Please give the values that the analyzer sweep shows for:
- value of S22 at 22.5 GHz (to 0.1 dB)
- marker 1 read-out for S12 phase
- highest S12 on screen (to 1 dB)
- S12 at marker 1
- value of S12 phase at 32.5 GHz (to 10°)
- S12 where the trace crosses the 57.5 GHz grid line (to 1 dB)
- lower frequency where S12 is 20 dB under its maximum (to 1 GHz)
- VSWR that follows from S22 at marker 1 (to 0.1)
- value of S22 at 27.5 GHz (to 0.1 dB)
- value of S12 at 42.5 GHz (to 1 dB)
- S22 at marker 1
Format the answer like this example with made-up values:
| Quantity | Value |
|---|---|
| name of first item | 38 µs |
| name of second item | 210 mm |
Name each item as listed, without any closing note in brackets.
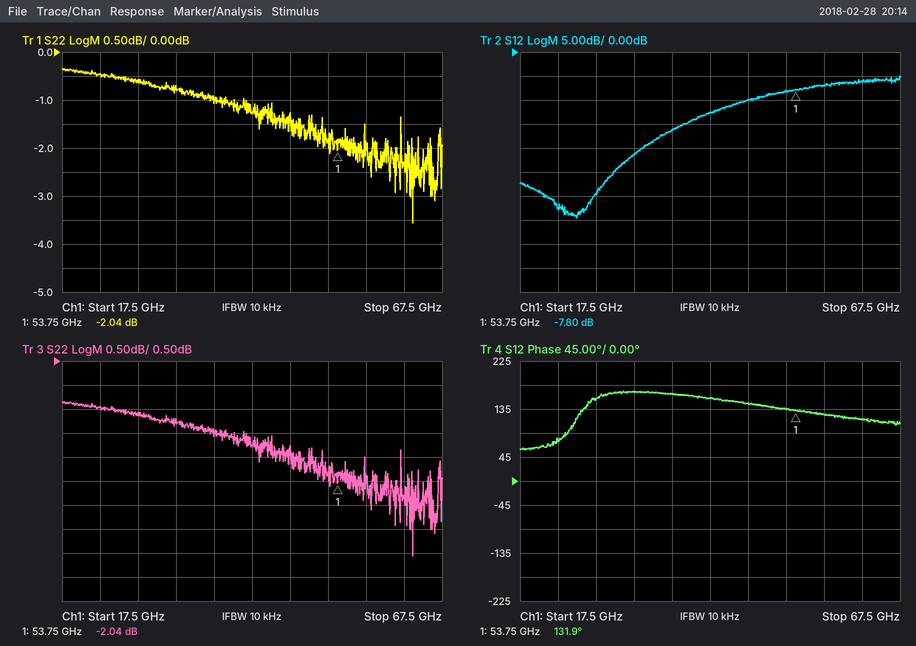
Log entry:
| Quantity | Value |
|---|---|
| value of S22 at 22.5 GHz | -0.5 dB |
| marker 1 read-out for S12 phase | 131.9° |
| highest S12 on screen | -5 dB |
| S12 at marker 1 | -7.80 dB |
| value of S12 phase at 32.5 GHz | 170° |
| S12 where the trace crosses the 57.5 GHz grid line | -7 dB |
| lower frequency where S12 is 20 dB under its maximum | 30 GHz |
| VSWR that follows from S22 at marker 1 | 8.6 |
| value of S22 at 27.5 GHz | -0.6 dB |
| value of S12 at 42.5 GHz | -13 dB |
| S22 at marker 1 | -2.04 dB |
